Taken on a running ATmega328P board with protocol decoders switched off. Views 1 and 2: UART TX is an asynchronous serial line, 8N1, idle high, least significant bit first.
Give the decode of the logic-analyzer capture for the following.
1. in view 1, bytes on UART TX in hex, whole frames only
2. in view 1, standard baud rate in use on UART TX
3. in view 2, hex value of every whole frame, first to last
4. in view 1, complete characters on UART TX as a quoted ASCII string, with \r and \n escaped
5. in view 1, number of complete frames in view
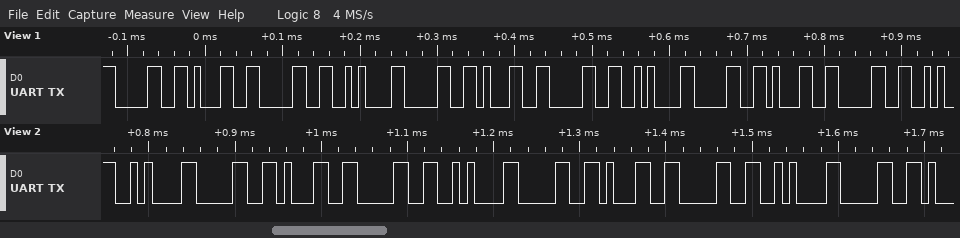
30 31 30 0A 30 31 30 0A 30 31 30
115200 baud
0x0A 0x30 0x31 0x30 0x0A 0x30 0x31 0x30 0x0A 0x30
"010\n010\n010"
11
